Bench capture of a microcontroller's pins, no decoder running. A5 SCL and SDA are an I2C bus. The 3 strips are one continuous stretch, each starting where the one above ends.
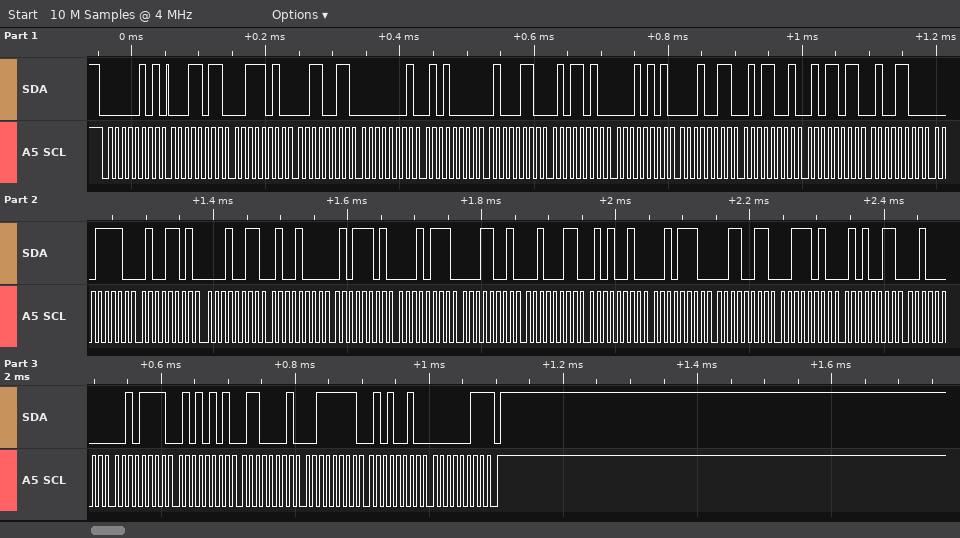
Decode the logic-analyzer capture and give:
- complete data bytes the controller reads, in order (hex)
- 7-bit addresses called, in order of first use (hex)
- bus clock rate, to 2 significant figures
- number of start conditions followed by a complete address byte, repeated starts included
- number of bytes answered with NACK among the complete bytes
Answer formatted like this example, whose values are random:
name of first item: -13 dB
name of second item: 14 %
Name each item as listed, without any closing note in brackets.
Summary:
complete data bytes the controller reads, in order: 1B 3A 33 01 50 46 5A 15 13 59 5B 4C 1E 4D 13 48 5D 17 19 23 52 2E 33 3A 53 20 2F 55 61 3F 52 03
7-bit addresses called, in order of first use: 0x02
bus clock rate, to 2 significant figures: 100 kHz
number of start conditions followed by a complete address byte, repeated starts included: 1
number of bytes answered with NACK among the complete bytes: 1
